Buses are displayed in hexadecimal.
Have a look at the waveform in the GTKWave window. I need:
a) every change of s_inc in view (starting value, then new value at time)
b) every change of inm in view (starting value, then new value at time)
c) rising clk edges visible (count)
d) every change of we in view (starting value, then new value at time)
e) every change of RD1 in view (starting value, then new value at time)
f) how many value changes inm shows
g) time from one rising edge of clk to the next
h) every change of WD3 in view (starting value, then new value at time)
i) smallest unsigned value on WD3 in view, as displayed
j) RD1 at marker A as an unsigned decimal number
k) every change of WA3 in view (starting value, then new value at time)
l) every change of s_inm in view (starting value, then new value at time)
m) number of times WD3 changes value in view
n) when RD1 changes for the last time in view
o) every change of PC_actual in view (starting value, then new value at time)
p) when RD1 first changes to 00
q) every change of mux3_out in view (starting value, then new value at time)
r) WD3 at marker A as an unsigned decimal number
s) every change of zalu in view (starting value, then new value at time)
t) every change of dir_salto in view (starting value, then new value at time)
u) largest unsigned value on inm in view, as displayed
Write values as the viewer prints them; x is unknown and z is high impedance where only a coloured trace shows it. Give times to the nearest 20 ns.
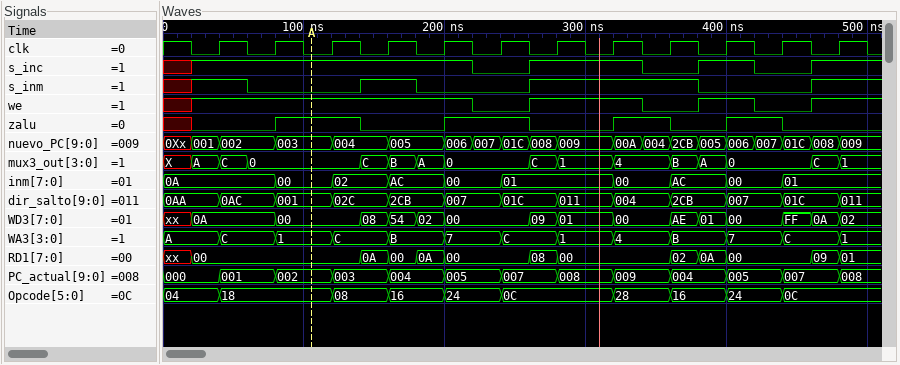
x, 1 at 20 ns, 0 at 220 ns, 1 at 260 ns, 0 at 340 ns, 1 at 380 ns, 0 at 420 ns, 1 at 460 ns
0A, 00 at 80 ns, 02 at 120 ns, AC at 160 ns, 00 at 200 ns, 01 at 240 ns, 00 at 320 ns, AC at 360 ns, 00 at 400 ns, 01 at 440 ns
12
x, 1 at 20 ns, 0 at 220 ns, 1 at 260 ns, 0 at 340 ns, 1 at 380 ns, 0 at 420 ns, 1 at 460 ns
xx, 00 at 20 ns, 0A at 140 ns, 00 at 160 ns, 0A at 180 ns, 00 at 200 ns, 08 at 260 ns, 00 at 280 ns, 02 at 360 ns, 0A at 380 ns, 00 at 400 ns, 09 at 460 ns, 01 at 480 ns
9
40 ns
xx, 0A at 20 ns, 00 at 80 ns, 08 at 140 ns, 54 at 160 ns, 02 at 180 ns, 00 at 200 ns, 09 at 260 ns, 01 at 280 ns, 00 at 320 ns, AE at 360 ns, 01 at 380 ns, 00 at 400 ns, FF at 440 ns, 0A at 460 ns, 02 at 480 ns
00
0
A, C at 40 ns, 1 at 80 ns, C at 120 ns, B at 160 ns, 7 at 200 ns, C at 240 ns, 1 at 280 ns, 4 at 320 ns, B at 360 ns, 7 at 400 ns, C at 440 ns, 1 at 480 ns
x, 1 at 20 ns, 0 at 60 ns, 1 at 140 ns, 0 at 180 ns, 1 at 260 ns, 0 at 380 ns, 1 at 460 ns
15
480 ns
000, 001 at 40 ns, 002 at 80 ns, 003 at 120 ns, 004 at 160 ns, 005 at 200 ns, 007 at 240 ns, 008 at 280 ns, 009 at 320 ns, 004 at 360 ns, 005 at 400 ns, 007 at 440 ns, 008 at 480 ns
20 ns
X, A at 20 ns, C at 40 ns, 0 at 60 ns, C at 140 ns, B at 160 ns, A at 180 ns, 0 at 200 ns, C at 260 ns, 1 at 280 ns, 4 at 320 ns, B at 360 ns, A at 380 ns, 0 at 400 ns, C at 460 ns, 1 at 480 ns
0
x, 0 at 20 ns, 1 at 80 ns, 0 at 140 ns, 1 at 200 ns, 0 at 260 ns, 1 at 320 ns, 0 at 360 ns, 1 at 400 ns, 0 at 440 ns
0AA, 0AC at 40 ns, 001 at 80 ns, 02C at 120 ns, 2CB at 160 ns, 007 at 200 ns, 01C at 240 ns, 011 at 280 ns, 004 at 320 ns, 2CB at 360 ns, 007 at 400 ns, 01C at 440 ns, 011 at 480 ns
AC
